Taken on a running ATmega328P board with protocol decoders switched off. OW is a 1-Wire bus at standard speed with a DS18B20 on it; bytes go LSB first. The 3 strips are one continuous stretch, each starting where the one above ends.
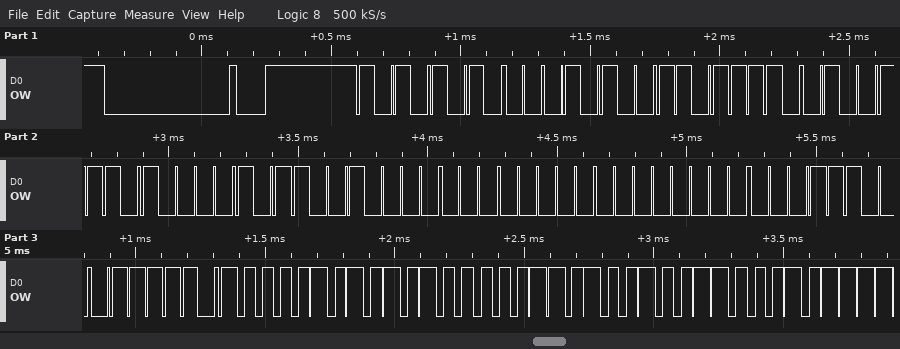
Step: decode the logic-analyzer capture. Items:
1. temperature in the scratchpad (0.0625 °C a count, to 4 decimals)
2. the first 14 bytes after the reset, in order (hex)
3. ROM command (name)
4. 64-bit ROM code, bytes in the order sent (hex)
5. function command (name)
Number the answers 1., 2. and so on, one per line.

1. 85.0000 °C
2. 55 28 7B 72 A1 09 00 00 38 BE 50 05 4B 46
3. Match ROM
4. 28 7B 72 A1 09 00 00 38
5. Read Scratchpad
